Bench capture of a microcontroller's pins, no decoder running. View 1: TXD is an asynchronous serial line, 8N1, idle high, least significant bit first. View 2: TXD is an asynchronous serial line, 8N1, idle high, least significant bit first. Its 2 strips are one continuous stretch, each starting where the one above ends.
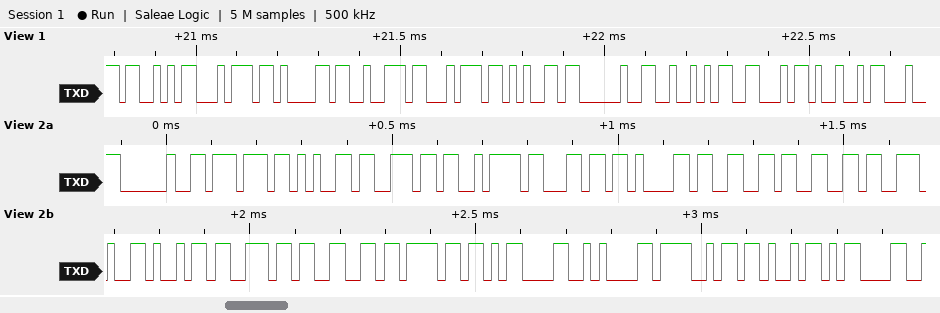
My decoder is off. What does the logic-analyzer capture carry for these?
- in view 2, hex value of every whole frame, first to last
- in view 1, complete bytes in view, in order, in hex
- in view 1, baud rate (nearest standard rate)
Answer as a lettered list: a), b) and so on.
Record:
a) 20 77 65 6E 7A 6C 61 66 66 2E 69 6E 66 6F 0D 0A 4F 4B 0D
b) 53 74 61 72 74 65 20 52 46 49
c) 57600 baud
